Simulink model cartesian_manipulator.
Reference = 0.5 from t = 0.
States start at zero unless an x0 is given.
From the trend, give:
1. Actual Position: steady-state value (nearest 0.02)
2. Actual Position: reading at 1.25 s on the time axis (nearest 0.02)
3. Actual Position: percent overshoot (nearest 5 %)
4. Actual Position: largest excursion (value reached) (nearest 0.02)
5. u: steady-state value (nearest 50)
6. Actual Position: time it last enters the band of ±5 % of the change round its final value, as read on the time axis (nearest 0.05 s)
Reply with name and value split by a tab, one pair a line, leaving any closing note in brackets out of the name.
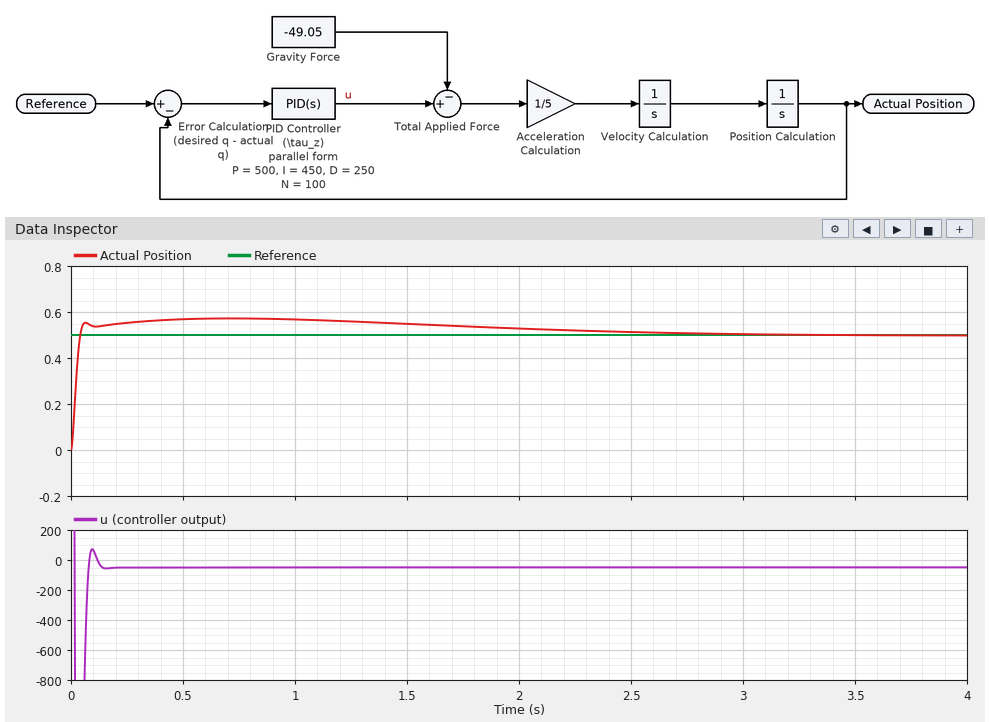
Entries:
Actual Position: steady-state value	0.50
Actual Position: reading at 1.25 s on the time axis	0.56
Actual Position: percent overshoot	15 %
Actual Position: largest excursion (value reached)	0.58
u: steady-state value	-50
Actual Position: time it last enters the band of ±5 % of the change round its final value, as read on the time axis	2.10 s
